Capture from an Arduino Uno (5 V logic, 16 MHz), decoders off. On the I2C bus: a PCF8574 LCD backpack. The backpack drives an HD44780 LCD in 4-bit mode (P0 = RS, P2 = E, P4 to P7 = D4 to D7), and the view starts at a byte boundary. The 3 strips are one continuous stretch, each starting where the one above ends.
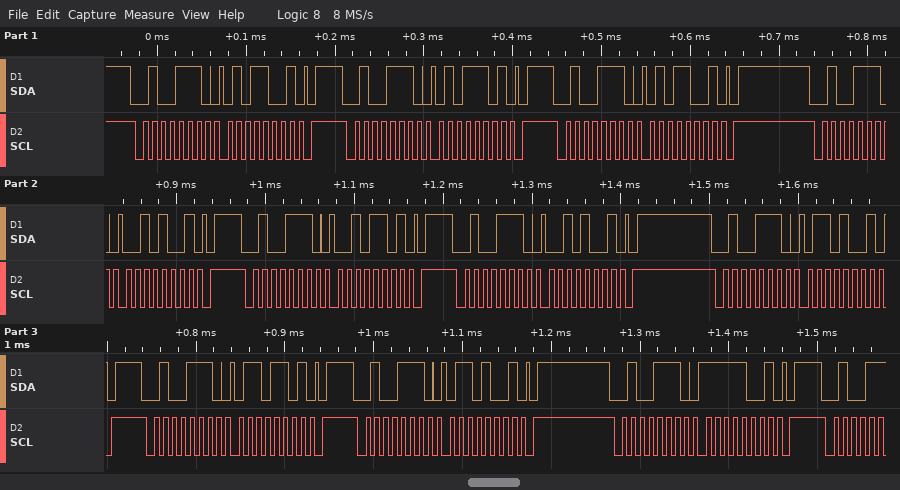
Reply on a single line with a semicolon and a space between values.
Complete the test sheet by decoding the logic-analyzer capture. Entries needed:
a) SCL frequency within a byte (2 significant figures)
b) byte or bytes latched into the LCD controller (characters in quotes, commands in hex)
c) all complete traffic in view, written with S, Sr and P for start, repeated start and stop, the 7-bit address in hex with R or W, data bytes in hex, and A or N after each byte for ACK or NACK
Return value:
100 kHz; 'R'; S 27W A 59 A P S 27W A 5D A P S 27W A 59 A P S 27W A 29 A P S 27W A 2D A P S 27W A 29 A P S 27W A 69 A P S 27W A 6D A P S 27W A 69 A P S 27W A F9 A P
